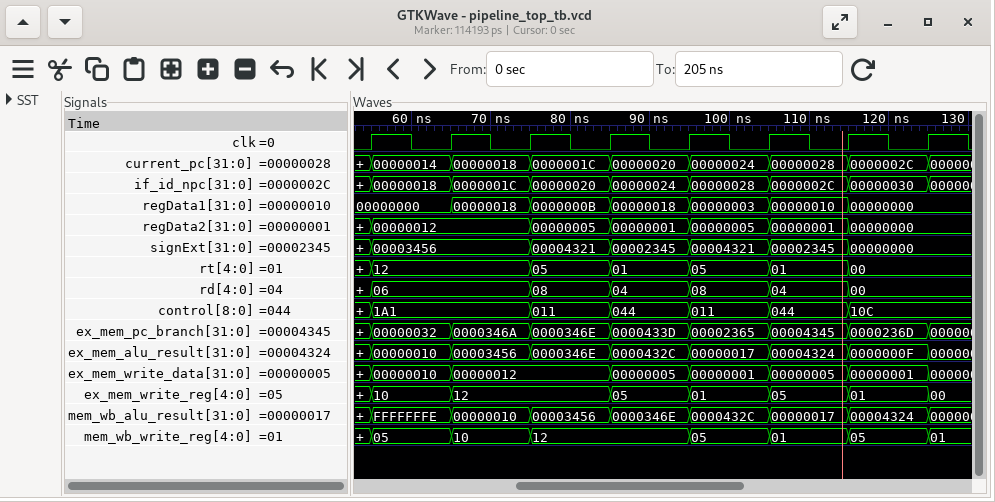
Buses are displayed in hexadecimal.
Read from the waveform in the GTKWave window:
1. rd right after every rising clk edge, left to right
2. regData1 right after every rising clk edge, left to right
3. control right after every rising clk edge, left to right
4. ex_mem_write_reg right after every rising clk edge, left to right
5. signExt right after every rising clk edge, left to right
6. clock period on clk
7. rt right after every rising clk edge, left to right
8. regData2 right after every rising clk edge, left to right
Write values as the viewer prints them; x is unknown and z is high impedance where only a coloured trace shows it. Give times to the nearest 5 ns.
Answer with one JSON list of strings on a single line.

["06, 06, 08, 04, 08, 04, 00, 00", "00000000, 00000018, 0000000B, 00000018, 00000003, 00000010, 00000000, 00000000", "1A1, 1A1, 011, 044, 011, 044, 10C, 10C", "10, 12, 12, 05, 01, 05, 01, 00", "00003456, 00003456, 00004321, 00002345, 00004321, 00002345, 00000000, 00000000", "10 ns", "12, 12, 05, 01, 05, 01, 00, 00", "00000012, 00000012, 00000005, 00000001, 00000005, 00000001, 00000000, 00000000"]
